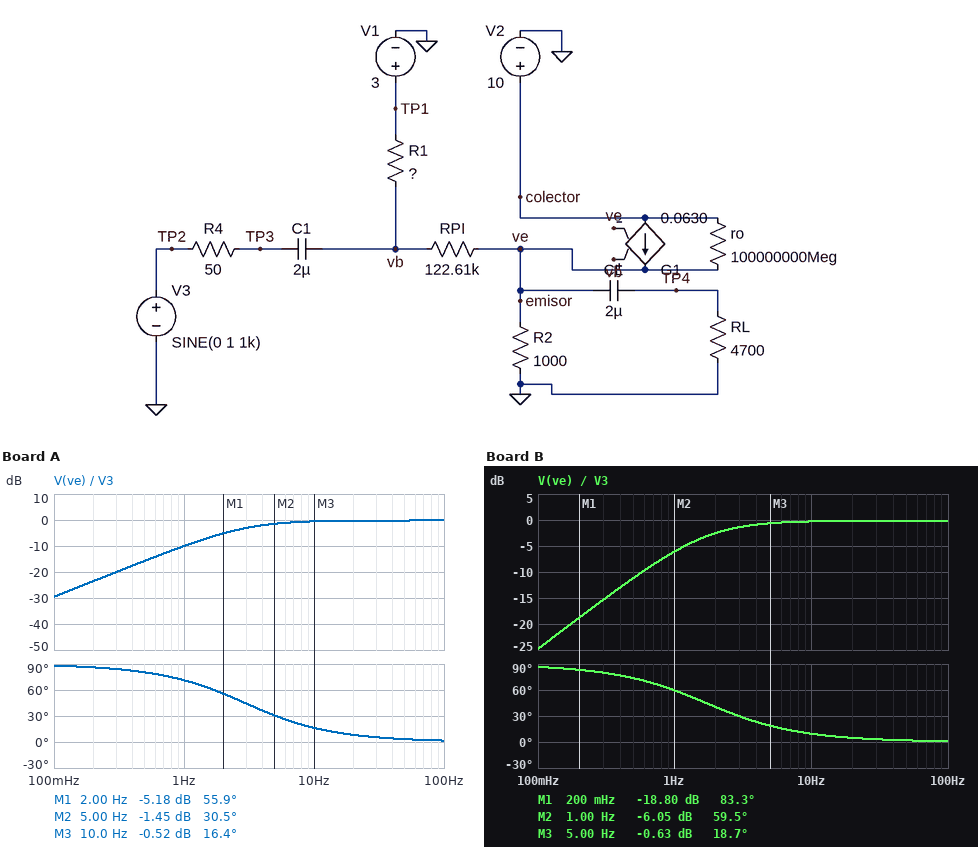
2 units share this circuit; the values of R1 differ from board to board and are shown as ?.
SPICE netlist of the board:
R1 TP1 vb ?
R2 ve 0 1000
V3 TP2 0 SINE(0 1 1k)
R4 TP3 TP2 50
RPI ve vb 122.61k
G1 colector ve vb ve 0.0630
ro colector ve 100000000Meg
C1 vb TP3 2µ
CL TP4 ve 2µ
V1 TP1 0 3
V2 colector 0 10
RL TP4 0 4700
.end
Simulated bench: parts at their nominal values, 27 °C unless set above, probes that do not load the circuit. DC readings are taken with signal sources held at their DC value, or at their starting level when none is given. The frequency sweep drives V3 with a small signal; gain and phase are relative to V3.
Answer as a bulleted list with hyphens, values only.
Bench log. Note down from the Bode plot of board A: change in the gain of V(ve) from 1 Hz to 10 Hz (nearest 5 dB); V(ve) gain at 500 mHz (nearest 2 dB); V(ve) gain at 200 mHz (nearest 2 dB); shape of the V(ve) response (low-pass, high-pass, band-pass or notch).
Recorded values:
- 10 dB
- -16 dB
- -24 dB
- high-pass
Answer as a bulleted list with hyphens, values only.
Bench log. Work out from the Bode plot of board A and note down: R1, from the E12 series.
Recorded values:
- 27 kΩ
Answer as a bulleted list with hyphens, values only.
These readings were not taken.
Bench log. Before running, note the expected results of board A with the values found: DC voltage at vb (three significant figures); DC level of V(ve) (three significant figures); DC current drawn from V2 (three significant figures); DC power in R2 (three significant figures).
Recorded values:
- 2.99 V
- 2.94 V
- 2.94 mA
- 8.66 mW
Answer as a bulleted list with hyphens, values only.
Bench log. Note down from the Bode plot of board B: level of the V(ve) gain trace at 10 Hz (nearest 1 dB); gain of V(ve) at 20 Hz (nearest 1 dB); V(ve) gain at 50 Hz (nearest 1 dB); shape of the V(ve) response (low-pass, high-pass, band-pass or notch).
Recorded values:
- 0 dB
- 0 dB
- 0 dB
- high-pass
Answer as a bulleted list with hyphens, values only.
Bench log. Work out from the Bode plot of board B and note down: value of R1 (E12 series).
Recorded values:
- 47 kΩ
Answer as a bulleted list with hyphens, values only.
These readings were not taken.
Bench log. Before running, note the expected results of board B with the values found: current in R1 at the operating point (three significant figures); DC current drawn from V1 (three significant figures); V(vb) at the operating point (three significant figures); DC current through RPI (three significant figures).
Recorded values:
- 380 nA
- 380 nA
- 2.98 V
- 380 nA
